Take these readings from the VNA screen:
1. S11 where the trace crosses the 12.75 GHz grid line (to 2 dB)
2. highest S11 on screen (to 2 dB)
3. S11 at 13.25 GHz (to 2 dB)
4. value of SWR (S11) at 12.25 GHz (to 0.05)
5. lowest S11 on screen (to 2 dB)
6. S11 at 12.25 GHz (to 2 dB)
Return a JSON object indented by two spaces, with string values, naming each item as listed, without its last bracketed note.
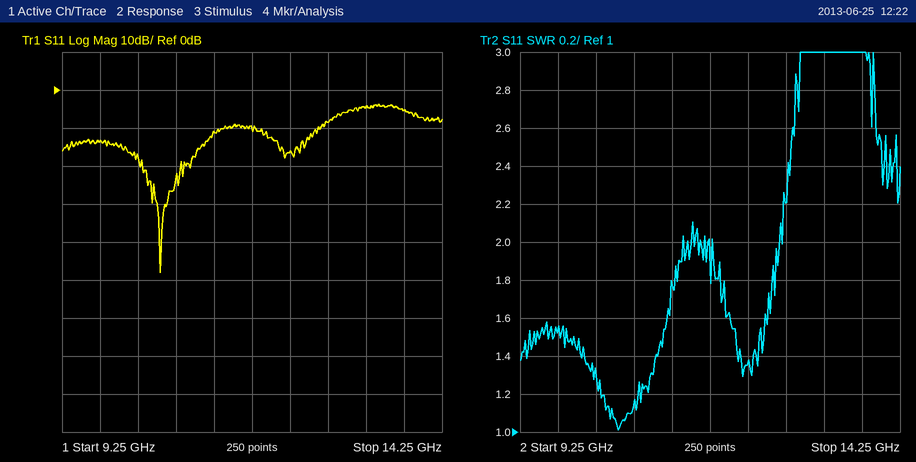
{
  "S11 where the trace crosses the 12.75 GHz grid line": "-8 dB",
  "highest S11 on screen": "-4 dB",
  "S11 at 13.25 GHz": "-4 dB",
  "value of SWR (S11) at 12.25 GHz": "1.35",
  "lowest S11 on screen": "-48 dB",
  "S11 at 12.25 GHz": "-16 dB"
}
